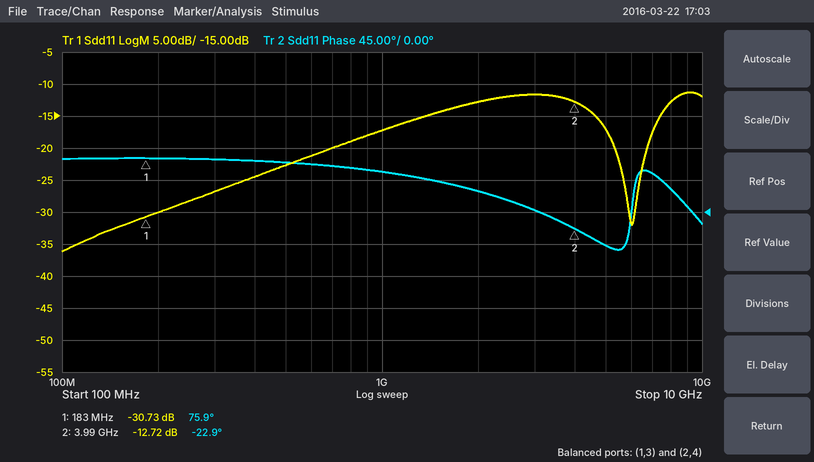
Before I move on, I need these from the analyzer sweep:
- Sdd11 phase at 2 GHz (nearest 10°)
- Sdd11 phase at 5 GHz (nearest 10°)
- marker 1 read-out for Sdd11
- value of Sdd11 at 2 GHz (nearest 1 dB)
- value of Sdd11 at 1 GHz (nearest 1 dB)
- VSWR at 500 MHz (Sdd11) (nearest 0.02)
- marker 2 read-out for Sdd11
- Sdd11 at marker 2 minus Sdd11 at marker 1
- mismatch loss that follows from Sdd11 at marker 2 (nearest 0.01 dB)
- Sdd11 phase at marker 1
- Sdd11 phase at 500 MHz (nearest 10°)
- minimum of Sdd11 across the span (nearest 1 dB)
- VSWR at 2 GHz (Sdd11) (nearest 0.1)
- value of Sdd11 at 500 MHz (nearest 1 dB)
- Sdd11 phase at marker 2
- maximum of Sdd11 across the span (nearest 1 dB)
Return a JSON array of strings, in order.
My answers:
["30°", "-50°", "-30.73 dB", "-13 dB", "-17 dB", "1.16", "-12.72 dB", "18.01 dB", "0.24 dB", "75.9°", "70°", "-36 dB", "1.6", "-23 dB", "-22.9°", "-11 dB"]
